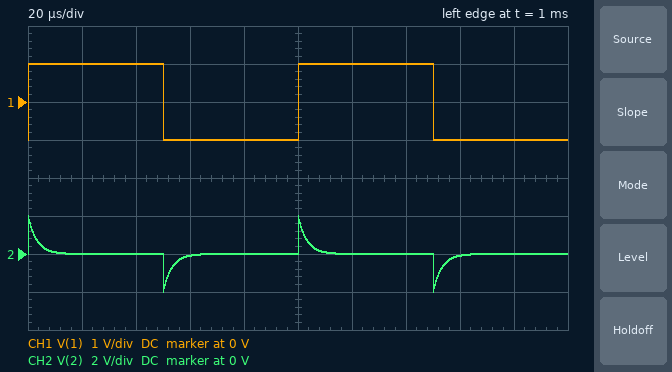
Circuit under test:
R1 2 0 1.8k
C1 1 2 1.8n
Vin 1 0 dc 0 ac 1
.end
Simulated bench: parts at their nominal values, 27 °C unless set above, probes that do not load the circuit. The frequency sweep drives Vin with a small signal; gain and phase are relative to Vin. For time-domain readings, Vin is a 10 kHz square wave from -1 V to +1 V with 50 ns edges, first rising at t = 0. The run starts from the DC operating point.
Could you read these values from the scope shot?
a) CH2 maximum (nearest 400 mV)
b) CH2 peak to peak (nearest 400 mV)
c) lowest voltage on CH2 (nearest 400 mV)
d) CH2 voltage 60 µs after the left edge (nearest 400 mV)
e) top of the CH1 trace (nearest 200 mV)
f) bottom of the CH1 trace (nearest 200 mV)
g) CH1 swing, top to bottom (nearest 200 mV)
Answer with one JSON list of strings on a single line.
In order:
["2.0 V", "4.0 V", "-2.0 V", "0 V", "1.0 V", "-1.0 V", "2.0 V"]
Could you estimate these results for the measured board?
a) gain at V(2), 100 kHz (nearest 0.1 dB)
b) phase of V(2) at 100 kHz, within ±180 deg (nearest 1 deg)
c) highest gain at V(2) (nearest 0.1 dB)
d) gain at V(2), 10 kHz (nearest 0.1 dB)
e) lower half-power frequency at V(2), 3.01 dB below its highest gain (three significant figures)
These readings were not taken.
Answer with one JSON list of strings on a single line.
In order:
["-0.9 dB", "26 deg", "0 dB", "-14.0 dB", "49.1 kHz"]
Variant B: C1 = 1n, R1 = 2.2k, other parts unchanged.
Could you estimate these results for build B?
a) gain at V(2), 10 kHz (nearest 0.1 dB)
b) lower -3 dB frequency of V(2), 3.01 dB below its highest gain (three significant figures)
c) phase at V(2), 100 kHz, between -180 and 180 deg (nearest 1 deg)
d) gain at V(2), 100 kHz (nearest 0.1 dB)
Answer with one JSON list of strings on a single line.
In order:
["-17.3 dB", "72.3 kHz", "36 deg", "-1.8 dB"]
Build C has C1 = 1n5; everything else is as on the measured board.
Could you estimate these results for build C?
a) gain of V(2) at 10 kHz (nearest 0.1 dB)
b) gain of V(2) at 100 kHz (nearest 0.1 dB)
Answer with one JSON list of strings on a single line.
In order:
["-15.5 dB", "-1.3 dB"]
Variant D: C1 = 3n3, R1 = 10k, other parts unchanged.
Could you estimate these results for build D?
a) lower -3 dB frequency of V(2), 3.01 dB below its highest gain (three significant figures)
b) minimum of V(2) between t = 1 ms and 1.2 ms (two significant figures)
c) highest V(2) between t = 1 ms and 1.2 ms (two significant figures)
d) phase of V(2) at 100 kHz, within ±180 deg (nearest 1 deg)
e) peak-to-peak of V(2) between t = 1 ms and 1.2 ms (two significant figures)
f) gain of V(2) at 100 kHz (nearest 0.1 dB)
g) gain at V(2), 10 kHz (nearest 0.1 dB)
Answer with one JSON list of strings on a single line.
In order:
["4.82 kHz", "-1.6 V", "1.6 V", "3 deg", "3.3 V", "0 dB", "-0.9 dB"]
